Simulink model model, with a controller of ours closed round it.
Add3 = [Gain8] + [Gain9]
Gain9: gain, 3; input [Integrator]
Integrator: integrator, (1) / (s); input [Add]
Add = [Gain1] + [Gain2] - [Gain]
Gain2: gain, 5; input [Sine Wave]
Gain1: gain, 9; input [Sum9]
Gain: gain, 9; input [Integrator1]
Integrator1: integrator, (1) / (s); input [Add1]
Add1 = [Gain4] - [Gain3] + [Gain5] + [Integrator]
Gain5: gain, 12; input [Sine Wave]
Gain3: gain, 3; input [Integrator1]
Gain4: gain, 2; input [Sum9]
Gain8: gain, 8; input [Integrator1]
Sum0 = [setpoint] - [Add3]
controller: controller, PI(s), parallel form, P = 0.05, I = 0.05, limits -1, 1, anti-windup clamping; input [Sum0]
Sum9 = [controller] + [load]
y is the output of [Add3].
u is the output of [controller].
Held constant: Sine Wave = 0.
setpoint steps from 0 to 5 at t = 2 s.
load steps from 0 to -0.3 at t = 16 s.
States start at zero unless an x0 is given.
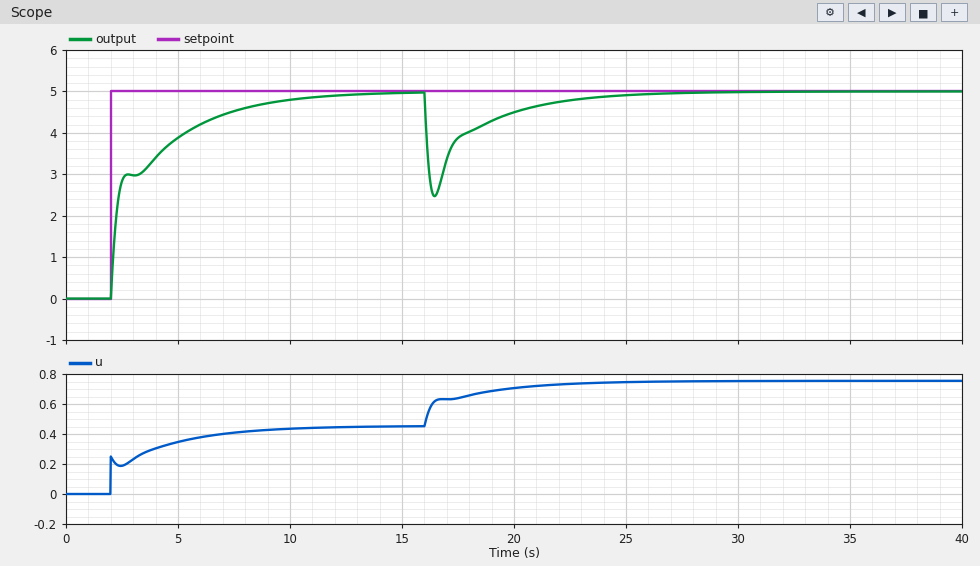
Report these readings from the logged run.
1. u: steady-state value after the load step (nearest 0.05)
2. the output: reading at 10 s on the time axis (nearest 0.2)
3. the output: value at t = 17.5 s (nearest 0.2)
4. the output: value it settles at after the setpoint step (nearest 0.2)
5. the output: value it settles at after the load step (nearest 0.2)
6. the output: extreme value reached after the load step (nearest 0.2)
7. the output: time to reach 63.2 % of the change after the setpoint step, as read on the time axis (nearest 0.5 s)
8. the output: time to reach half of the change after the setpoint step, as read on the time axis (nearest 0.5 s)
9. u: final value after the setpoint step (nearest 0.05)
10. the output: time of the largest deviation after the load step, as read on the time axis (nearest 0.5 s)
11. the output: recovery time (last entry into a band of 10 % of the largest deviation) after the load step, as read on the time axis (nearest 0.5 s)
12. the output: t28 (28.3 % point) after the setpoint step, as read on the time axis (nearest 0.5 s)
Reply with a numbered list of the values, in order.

1. 0.75
2. 4.8
3. 3.8
4. 5.0
5. 5.0
6. 2.4
7. 3.5 s
8. 2.5 s
9. 0.45
10. 16.5 s
11. 22.0 s
12. 2.0 s
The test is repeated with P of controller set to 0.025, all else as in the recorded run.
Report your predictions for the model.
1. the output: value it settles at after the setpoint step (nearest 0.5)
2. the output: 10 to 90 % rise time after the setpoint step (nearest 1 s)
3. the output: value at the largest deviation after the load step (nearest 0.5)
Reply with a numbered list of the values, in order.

1. 5.0
2. 5 s
3. 2.0
